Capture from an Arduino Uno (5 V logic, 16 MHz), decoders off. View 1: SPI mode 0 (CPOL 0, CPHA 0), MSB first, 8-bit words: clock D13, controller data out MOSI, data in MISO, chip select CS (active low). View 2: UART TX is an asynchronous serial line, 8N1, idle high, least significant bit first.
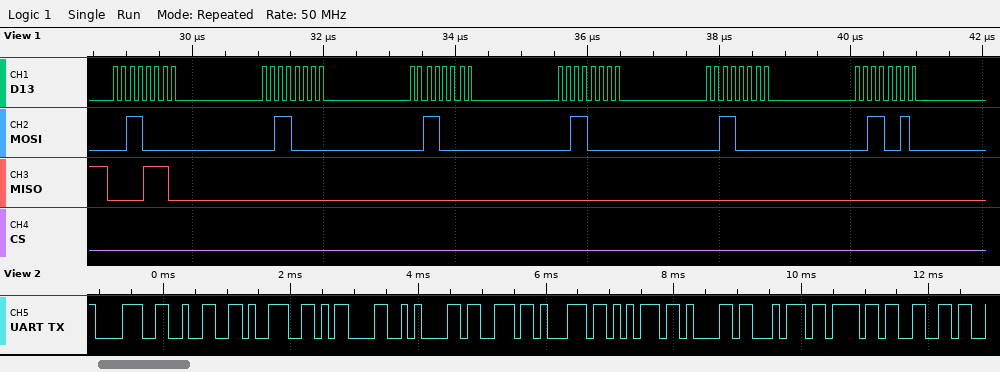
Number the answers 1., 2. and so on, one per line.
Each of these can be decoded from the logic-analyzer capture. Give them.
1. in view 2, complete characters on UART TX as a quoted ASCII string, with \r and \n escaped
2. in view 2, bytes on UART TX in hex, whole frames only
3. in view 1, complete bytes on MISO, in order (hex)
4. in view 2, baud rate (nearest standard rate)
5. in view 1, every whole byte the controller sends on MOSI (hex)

1. "829\r\nsquatof"
2. 38 32 39 0D 0A 73 71 75 61 74 6F 66
3. 0x0E 0x00 0x00 0x00 0x00 0x00
4. 9600 baud
5. 0x30 0x30 0x30 0x30 0x30 0x32
